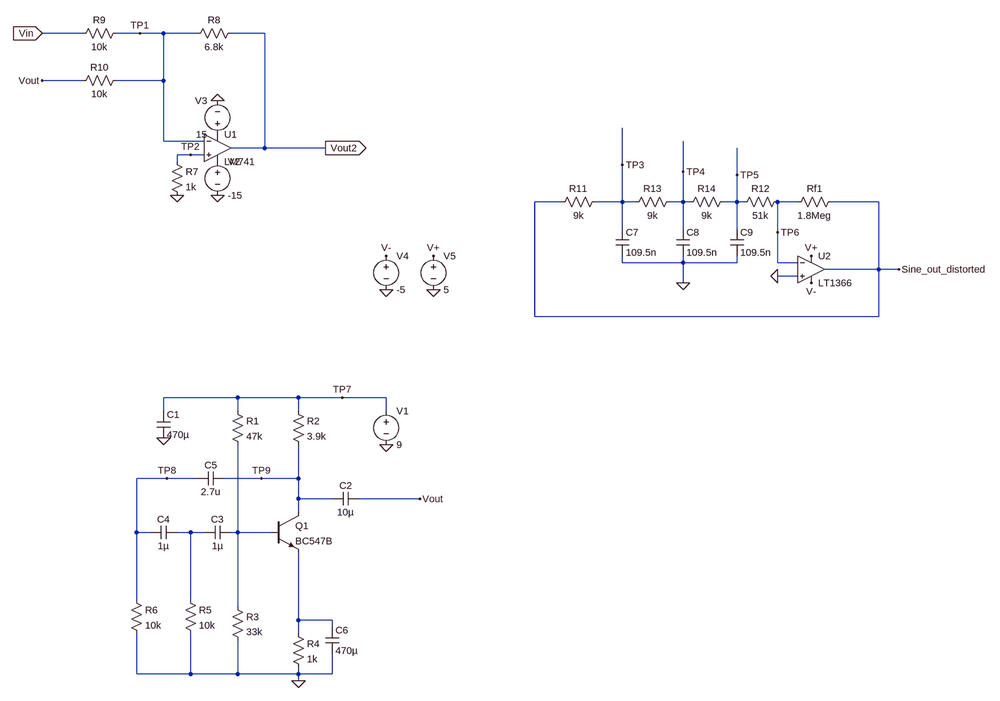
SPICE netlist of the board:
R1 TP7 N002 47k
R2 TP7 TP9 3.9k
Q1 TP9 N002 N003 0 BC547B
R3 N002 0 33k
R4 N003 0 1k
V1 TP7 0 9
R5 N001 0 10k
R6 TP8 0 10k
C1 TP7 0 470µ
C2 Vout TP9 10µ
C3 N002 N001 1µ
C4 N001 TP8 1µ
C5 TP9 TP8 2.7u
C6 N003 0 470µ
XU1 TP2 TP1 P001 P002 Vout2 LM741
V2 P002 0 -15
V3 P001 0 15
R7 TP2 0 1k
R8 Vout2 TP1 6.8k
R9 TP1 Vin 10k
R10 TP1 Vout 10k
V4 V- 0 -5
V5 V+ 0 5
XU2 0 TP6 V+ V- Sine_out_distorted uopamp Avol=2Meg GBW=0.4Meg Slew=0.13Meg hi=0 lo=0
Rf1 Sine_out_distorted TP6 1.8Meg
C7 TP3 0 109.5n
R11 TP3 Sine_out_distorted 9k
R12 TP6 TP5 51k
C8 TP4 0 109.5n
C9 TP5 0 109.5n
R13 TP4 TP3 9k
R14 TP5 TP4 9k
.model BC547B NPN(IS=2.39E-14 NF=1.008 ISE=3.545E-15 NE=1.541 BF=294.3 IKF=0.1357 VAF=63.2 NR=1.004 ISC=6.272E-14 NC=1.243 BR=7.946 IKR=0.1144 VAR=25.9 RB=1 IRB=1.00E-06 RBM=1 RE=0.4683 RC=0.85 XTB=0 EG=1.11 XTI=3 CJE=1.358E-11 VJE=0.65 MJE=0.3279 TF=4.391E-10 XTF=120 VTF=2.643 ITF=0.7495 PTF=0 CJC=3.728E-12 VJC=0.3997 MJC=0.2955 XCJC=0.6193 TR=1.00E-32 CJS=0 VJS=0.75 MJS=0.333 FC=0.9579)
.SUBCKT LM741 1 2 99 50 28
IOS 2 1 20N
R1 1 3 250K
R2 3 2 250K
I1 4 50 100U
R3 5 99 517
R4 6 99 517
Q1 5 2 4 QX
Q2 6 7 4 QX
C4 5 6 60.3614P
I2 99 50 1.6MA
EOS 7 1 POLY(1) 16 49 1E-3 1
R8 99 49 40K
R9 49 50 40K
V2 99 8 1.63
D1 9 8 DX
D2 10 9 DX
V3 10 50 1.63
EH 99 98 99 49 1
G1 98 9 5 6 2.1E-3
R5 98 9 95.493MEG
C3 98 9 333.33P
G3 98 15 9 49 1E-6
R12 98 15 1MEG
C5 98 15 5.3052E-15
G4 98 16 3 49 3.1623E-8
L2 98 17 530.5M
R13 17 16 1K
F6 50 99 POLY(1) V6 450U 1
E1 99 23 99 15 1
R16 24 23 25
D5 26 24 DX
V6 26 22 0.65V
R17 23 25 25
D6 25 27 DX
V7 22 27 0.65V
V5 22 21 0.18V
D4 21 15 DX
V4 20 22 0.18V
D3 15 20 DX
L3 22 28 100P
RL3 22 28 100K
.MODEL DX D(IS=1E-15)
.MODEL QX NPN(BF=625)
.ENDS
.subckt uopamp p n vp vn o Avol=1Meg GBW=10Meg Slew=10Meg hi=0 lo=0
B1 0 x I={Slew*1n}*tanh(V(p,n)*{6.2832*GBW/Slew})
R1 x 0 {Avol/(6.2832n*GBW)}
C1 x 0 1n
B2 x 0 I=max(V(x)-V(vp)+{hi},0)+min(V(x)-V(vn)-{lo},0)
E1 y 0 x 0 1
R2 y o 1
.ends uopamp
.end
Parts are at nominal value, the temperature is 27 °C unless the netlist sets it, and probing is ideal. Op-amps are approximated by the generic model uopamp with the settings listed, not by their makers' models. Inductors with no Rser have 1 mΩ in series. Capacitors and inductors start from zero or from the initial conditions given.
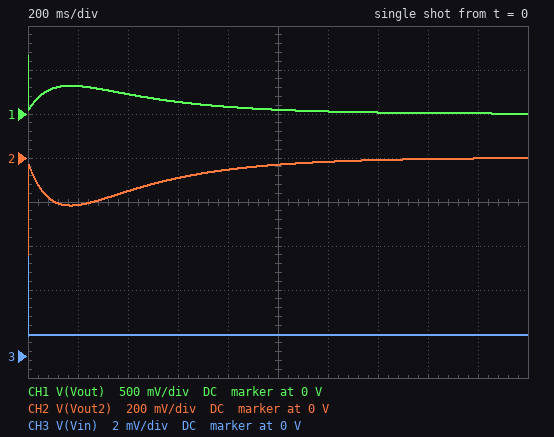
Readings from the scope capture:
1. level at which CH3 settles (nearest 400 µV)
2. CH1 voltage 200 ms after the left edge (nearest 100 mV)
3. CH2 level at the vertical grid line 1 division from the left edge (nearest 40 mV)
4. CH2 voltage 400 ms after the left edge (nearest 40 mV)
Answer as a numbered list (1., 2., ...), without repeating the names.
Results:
1. 800 µV
2. 300 mV
3. -200 mV
4. -160 mV
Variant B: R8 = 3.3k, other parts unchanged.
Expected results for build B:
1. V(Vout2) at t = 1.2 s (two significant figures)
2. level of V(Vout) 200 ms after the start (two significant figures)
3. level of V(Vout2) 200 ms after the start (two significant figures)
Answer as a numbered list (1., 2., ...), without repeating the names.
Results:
1. -7.8 mV
2. 320 mV
3. -100 mV
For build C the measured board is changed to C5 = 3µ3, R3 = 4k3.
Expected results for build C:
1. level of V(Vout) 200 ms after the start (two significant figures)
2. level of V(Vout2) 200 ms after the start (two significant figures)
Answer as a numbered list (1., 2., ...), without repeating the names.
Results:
1. 2.3 V
2. -1.6 V
